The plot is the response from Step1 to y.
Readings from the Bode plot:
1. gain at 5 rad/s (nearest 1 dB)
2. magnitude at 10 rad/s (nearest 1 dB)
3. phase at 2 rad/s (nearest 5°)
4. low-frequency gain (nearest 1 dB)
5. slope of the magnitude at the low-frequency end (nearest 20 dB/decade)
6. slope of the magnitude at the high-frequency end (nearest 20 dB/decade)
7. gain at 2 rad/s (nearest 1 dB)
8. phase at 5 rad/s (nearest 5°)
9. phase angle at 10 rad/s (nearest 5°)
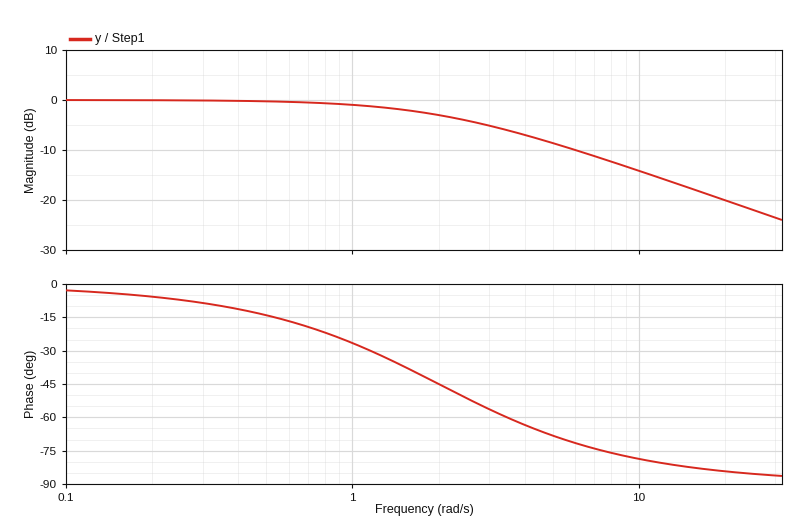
-9 dB
-14 dB
-45°
0 dB
0 dB/decade
-20 dB/decade
-3 dB
-70°
-80°
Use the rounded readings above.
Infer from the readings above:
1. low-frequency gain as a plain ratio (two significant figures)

1.0
